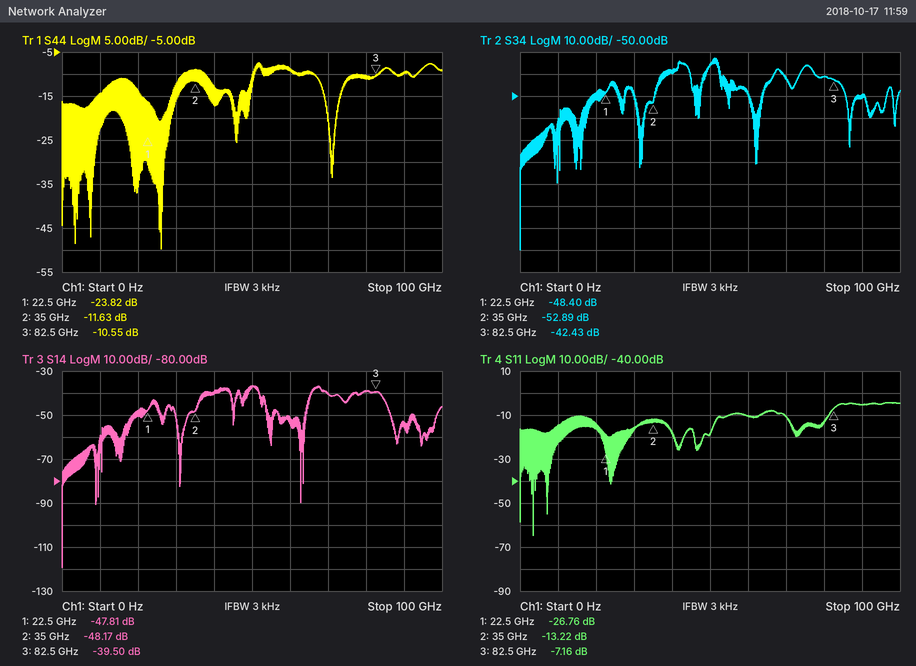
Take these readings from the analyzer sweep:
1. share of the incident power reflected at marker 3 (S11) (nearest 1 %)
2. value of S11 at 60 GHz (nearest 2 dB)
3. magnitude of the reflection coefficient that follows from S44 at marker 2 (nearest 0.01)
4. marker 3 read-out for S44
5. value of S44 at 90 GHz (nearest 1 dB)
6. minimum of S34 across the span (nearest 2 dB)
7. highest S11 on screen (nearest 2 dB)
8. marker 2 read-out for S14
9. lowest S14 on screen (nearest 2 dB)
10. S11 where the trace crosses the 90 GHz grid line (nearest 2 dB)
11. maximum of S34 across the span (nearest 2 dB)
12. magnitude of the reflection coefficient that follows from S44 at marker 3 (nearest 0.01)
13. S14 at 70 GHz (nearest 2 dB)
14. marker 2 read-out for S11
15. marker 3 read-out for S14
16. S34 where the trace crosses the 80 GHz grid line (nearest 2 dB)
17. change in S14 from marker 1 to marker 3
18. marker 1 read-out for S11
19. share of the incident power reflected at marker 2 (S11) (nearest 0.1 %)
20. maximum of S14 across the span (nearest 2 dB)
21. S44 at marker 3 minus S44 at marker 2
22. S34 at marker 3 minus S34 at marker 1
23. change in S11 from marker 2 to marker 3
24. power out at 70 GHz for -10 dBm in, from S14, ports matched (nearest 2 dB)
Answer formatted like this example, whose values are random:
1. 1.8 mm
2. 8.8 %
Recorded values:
1. 19 %
2. -10 dB
3. 0.26
4. -10.55 dB
5. -10 dB
6. -120 dB
7. -4 dB
8. -48.17 dB
9. -120 dB
10. -6 dB
11. -32 dB
12. 0.30
13. -40 dB
14. -13.22 dB
15. -39.50 dB
16. -42 dB
17. 8.31 dB
18. -26.76 dB
19. 4.8 %
20. -36 dB
21. 1.08 dB
22. 5.97 dB
23. 6.06 dB
24. -50 dBm
